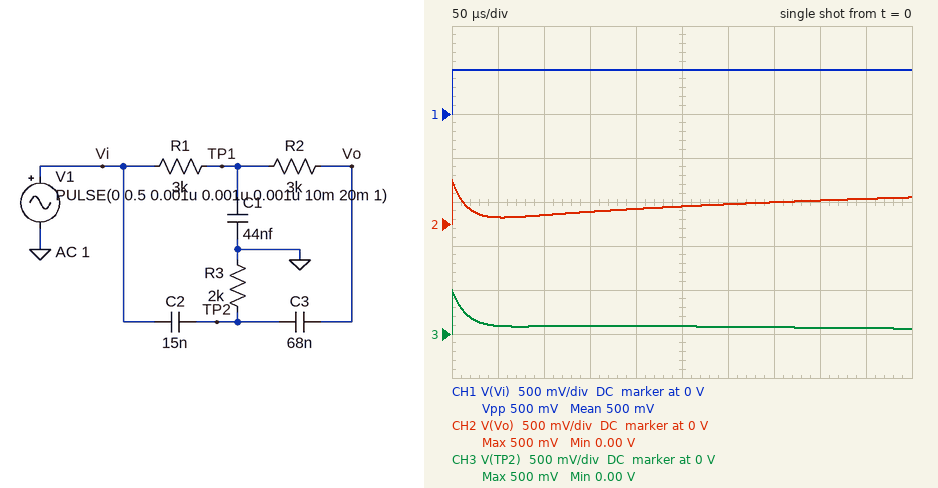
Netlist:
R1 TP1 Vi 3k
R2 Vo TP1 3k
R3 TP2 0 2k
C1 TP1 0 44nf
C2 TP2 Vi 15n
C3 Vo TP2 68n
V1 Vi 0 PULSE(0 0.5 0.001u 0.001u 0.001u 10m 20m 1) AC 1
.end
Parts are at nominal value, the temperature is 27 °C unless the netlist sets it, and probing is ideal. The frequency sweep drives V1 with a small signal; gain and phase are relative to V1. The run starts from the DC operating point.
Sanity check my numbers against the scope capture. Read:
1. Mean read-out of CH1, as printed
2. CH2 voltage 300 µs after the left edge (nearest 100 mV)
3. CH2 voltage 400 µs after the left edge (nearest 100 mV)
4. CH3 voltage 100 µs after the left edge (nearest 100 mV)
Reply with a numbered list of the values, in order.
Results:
1. 500 mV
2. 200 mV
3. 300 mV
4. 100 mV
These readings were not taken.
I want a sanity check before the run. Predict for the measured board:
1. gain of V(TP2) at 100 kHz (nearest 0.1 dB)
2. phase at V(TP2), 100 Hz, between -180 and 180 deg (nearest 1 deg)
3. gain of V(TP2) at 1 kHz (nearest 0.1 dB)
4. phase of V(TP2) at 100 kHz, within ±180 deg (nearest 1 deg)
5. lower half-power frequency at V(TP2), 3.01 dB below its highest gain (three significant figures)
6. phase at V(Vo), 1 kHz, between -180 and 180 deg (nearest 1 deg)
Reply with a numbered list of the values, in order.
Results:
1. 0 dB
2. 69 deg
3. -12.5 dB
4. 5 deg
5. 10.2 kHz
6. -50 deg
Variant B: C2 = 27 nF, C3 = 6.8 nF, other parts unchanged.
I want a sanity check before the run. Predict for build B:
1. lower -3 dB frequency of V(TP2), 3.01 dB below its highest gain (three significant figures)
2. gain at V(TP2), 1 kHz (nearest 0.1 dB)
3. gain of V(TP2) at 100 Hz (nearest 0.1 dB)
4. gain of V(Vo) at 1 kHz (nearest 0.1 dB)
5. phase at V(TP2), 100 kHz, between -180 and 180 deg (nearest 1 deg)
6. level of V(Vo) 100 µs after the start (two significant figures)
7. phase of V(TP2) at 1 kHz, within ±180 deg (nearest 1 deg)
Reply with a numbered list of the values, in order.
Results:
1. 4.37 kHz
2. -9.2 dB
3. -27.5 dB
4. -3.8 dB
5. 3 deg
6. 180 mV
7. 61 deg
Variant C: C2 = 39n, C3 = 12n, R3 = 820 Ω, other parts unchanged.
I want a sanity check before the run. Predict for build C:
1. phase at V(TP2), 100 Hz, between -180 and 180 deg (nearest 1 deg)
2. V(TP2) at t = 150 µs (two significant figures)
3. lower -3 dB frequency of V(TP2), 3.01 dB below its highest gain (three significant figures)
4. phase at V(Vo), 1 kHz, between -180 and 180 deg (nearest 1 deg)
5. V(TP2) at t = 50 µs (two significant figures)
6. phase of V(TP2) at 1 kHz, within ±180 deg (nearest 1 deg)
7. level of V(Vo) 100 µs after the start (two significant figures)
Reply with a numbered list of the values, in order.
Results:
1. 87 deg
2. 26 mV
3. 6.76 kHz
4. -58 deg
5. 110 mV
6. 67 deg
7. 140 mV
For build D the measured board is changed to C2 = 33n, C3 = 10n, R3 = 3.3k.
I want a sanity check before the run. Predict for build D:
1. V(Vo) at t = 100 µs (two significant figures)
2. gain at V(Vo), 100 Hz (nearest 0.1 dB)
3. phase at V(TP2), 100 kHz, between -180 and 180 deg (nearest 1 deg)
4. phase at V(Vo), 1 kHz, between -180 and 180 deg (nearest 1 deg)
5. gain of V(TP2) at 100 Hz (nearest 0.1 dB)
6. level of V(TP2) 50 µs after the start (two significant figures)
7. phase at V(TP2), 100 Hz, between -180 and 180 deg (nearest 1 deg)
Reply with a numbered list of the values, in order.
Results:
1. 180 mV
2. -0.1 dB
3. 2 deg
4. -48 deg
5. -21.1 dB
6. 280 mV
7. 83 deg
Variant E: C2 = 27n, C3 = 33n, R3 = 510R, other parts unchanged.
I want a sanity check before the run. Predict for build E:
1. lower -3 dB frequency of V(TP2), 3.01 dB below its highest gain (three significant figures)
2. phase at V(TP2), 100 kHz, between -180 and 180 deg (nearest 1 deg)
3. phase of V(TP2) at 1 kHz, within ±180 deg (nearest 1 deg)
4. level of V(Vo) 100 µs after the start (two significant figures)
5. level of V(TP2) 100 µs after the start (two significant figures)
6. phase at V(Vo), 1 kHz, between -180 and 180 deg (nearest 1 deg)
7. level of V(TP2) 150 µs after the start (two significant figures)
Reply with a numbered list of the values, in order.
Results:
1. 14.1 kHz
2. 8 deg
3. 56 deg
4. 88 mV
5. 23 mV
6. -75 deg
7. 21 mV
